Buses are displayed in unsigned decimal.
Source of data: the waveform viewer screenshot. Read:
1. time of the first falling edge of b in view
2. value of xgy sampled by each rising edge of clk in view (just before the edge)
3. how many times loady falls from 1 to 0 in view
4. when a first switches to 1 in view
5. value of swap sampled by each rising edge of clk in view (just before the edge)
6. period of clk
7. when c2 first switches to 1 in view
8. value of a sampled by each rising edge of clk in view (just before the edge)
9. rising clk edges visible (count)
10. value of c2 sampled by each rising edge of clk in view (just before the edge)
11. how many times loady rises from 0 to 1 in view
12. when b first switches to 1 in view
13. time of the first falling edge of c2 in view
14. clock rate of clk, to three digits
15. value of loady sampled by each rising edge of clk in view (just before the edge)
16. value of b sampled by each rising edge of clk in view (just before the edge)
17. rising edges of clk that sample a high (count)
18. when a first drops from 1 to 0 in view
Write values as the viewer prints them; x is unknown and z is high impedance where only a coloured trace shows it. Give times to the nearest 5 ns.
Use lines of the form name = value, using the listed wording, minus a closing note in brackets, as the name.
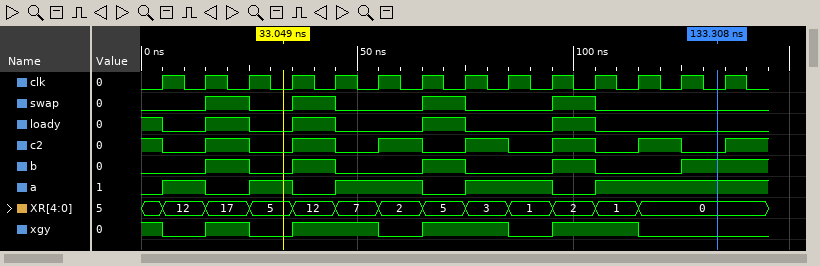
time of the first falling edge of b in view = 25 ns
value of xgy sampled by each rising edge of clk in view = 1 0 1 0 1 1 0 1 1 0 1 1 0 0
how many times loady falls from 1 to 0 in view = 5
when a first switches to 1 in view = 5 ns
value of swap sampled by each rising edge of clk in view = 0 0 1 0 1 0 0 1 0 0 1 0 0 0
period of clk = 10 ns
when c2 first switches to 1 in view = 15 ns
value of a sampled by each rising edge of clk in view = 0 1 0 1 0 1 1 0 1 1 0 1 1 1
rising clk edges visible = 14
value of c2 sampled by each rising edge of clk in view = 1 0 1 0 1 0 1 0 1 0 1 0 1 0
how many times loady rises from 0 to 1 in view = 4
when b first switches to 1 in view = 15 ns
time of the first falling edge of c2 in view = 5 ns
clock rate of clk, to three digits = 100 MHz
value of loady sampled by each rising edge of clk in view = 1 0 1 0 1 0 0 1 0 0 1 0 0 0
value of b sampled by each rising edge of clk in view = 0 0 1 0 1 0 0 1 0 0 1 0 0 1
rising edges of clk that sample a high = 9
when a first drops from 1 to 0 in view = 15 ns
